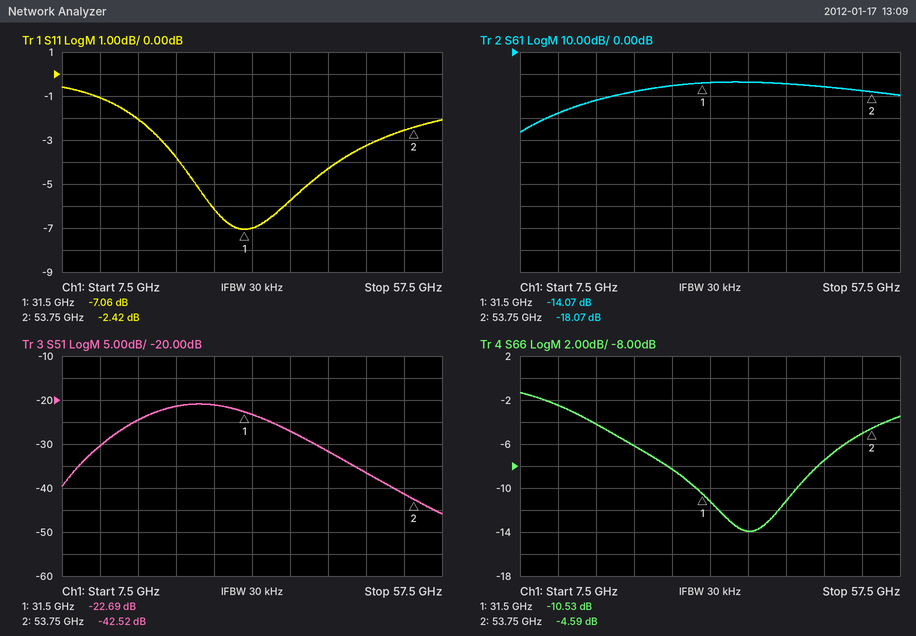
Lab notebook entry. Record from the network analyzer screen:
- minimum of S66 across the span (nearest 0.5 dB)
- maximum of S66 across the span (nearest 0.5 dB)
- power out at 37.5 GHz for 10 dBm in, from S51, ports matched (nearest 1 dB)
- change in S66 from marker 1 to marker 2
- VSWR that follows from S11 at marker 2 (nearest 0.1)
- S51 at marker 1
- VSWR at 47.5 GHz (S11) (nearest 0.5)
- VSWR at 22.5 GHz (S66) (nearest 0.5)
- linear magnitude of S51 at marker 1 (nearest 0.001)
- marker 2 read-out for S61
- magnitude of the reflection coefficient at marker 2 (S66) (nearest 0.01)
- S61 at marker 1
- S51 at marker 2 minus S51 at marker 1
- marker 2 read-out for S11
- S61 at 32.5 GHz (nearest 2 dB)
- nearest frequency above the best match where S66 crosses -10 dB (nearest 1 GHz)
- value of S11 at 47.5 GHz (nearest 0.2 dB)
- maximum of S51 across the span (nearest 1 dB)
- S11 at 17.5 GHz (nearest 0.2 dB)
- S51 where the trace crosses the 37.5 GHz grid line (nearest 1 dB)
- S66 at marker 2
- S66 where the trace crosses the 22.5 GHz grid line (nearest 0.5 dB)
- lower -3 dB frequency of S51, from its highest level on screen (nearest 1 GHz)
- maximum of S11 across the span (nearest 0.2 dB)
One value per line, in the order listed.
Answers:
-14.0 dB
-1.5 dB
-17 dBm
5.94 dB
7.2
-22.69 dB
5.5
3.0
0.073
-18.07 dB
0.59
-14.07 dB
-19.83 dB
-2.42 dB
-14 dB
44 GHz
-3.2 dB
-21 dB
-2.0 dB
-27 dB
-4.59 dB
-6.0 dB
18 GHz
-0.6 dB
